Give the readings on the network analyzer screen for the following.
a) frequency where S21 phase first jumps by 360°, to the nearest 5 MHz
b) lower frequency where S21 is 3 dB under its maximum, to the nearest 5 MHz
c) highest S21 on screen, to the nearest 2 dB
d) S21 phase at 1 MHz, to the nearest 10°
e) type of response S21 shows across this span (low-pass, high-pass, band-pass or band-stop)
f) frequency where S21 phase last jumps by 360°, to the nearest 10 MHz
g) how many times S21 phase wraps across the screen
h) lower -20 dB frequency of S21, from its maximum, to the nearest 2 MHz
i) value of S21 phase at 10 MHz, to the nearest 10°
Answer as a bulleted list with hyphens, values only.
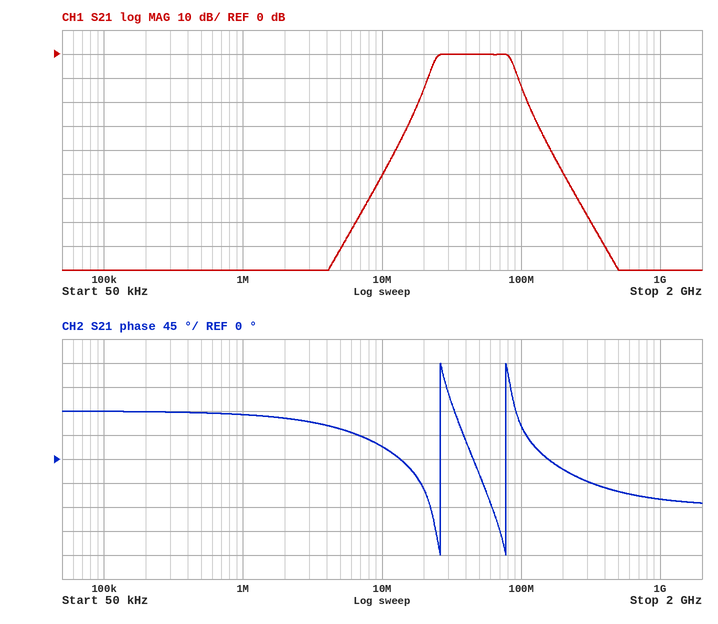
- 25 MHz
- 25 MHz
- 0 dB
- 80°
- band-pass
- 80 MHz
- 2
- 18 MHz
- 20°
